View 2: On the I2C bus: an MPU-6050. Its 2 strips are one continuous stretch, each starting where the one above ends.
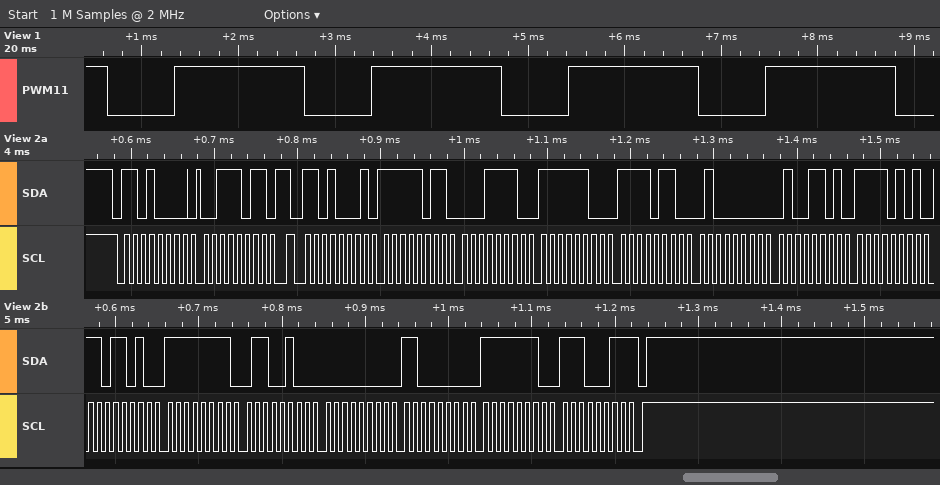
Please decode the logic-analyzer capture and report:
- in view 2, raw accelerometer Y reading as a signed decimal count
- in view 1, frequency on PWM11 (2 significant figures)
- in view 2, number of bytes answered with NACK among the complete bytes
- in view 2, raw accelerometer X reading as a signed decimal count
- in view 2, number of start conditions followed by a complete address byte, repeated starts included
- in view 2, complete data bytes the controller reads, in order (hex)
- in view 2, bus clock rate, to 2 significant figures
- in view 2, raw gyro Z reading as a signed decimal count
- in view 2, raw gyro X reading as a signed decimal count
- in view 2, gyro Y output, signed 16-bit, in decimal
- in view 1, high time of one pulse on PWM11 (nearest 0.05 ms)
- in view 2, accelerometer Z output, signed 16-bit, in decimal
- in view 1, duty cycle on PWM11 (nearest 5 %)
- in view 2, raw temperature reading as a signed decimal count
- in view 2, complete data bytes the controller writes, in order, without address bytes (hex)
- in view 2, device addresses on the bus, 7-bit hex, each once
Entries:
-778
490 Hz
1
-1250
2
FB 1E FC F6 40 4D F5 DA FF 64 00 C0 FE E3
100 kHz
-285
-156
192
1.35 ms
16461
65 %
-2598
3B
0x68
